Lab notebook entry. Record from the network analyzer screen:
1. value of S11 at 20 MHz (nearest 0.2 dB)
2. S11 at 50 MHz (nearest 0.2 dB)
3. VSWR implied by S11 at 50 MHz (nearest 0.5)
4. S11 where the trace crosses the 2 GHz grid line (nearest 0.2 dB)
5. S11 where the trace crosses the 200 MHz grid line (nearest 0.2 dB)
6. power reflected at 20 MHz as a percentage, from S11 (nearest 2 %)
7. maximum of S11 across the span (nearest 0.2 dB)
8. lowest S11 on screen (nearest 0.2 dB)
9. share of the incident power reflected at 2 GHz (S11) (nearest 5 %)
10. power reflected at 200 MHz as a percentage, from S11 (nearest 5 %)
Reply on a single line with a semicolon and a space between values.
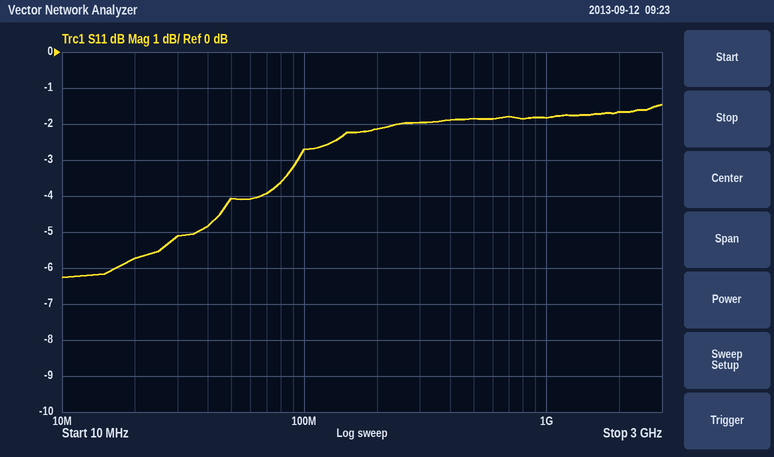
-5.8 dB; -4.0 dB; 4.5; -1.6 dB; -2.2 dB; 26 %; -1.4 dB; -6.2 dB; 70 %; 60 %
